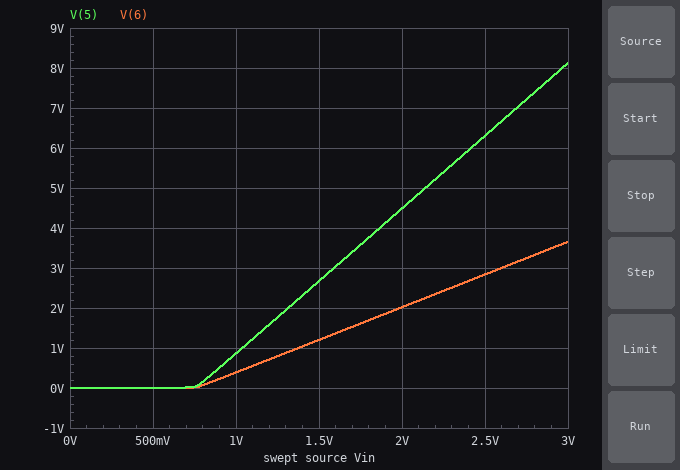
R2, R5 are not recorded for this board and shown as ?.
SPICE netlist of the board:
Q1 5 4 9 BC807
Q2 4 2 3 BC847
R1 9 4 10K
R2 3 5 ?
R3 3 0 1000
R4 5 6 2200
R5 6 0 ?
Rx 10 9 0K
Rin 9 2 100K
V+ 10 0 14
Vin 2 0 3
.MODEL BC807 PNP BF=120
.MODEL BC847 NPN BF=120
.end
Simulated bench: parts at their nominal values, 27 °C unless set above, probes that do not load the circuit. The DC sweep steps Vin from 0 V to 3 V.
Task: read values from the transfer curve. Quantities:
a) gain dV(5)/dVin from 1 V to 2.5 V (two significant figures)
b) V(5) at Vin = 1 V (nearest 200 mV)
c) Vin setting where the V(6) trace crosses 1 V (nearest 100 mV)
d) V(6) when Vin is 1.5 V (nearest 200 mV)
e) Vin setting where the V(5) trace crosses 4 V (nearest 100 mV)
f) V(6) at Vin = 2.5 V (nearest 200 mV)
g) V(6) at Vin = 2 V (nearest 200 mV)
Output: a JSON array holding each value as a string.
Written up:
["3.6 V/V", "800 mV", "1.4 V", "1.2 V", "1.9 V", "2.8 V", "2.0 V"]
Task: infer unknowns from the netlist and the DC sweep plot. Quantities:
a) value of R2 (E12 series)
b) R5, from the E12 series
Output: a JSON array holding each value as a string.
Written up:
["2.7 kΩ", "1.8 kΩ"]
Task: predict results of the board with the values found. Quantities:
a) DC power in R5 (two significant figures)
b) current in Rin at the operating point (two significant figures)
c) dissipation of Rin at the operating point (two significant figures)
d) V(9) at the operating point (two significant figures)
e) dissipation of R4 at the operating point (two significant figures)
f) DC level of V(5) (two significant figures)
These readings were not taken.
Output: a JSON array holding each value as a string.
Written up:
["7.4 mW", "110 µA", "1.2 mW", "14 V", "9.1 mW", "8.1 V"]
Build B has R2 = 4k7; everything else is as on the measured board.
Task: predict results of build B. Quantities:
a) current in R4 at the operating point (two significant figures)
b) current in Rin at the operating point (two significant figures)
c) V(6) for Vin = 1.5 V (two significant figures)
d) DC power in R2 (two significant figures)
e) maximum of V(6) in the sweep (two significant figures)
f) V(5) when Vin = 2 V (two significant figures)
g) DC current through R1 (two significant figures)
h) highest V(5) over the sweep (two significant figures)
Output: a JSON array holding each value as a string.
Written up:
["3.1 mA", "110 µA", "1.8 V", "22 mW", "5.6 V", "6.8 V", "82 µA", "12 V"]
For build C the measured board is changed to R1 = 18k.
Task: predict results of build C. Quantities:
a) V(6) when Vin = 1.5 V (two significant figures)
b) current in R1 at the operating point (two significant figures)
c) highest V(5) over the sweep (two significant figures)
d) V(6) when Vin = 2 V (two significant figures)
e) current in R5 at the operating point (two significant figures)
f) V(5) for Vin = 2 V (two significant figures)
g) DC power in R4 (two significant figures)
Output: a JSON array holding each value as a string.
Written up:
["1.3 V", "45 µA", "8.3 V", "2.1 V", "2.1 mA", "4.6 V", "9.4 mW"]
